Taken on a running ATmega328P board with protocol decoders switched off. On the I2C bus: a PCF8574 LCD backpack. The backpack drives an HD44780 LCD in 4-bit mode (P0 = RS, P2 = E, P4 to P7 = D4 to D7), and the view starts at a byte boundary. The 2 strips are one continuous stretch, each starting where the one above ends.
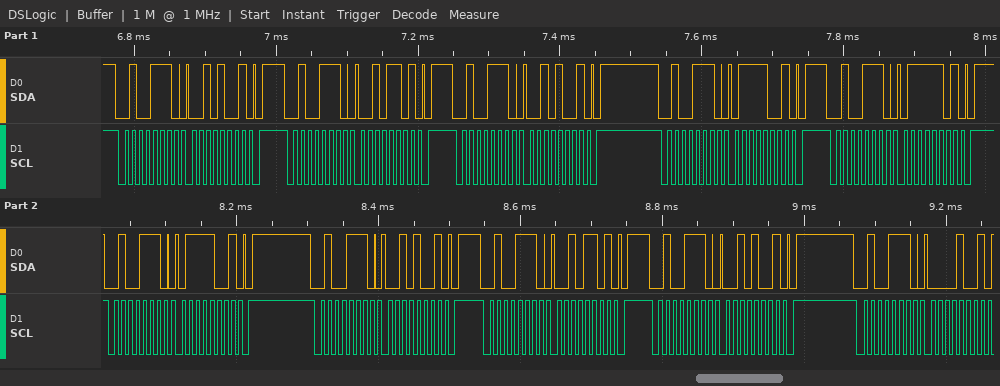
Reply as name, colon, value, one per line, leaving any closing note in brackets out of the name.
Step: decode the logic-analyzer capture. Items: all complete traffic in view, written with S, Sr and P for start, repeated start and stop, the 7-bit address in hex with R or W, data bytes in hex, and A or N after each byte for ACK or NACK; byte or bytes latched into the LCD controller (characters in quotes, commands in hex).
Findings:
all complete traffic in view, written with S, Sr and P for start, repeated start and stop, the 7-bit address in hex with R or W, data bytes in hex, and A or N after each byte for ACK or NACK: S 27W A 29 A P S 27W A 2D A P S 27W A 29 A P S 27W A 79 A P S 27W A 7D A P S 27W A 79 A P S 27W A 29 A P S 27W A 2D A P S 27W A 29 A P S 27W A 09 A
byte or bytes latched into the LCD controller: '''
